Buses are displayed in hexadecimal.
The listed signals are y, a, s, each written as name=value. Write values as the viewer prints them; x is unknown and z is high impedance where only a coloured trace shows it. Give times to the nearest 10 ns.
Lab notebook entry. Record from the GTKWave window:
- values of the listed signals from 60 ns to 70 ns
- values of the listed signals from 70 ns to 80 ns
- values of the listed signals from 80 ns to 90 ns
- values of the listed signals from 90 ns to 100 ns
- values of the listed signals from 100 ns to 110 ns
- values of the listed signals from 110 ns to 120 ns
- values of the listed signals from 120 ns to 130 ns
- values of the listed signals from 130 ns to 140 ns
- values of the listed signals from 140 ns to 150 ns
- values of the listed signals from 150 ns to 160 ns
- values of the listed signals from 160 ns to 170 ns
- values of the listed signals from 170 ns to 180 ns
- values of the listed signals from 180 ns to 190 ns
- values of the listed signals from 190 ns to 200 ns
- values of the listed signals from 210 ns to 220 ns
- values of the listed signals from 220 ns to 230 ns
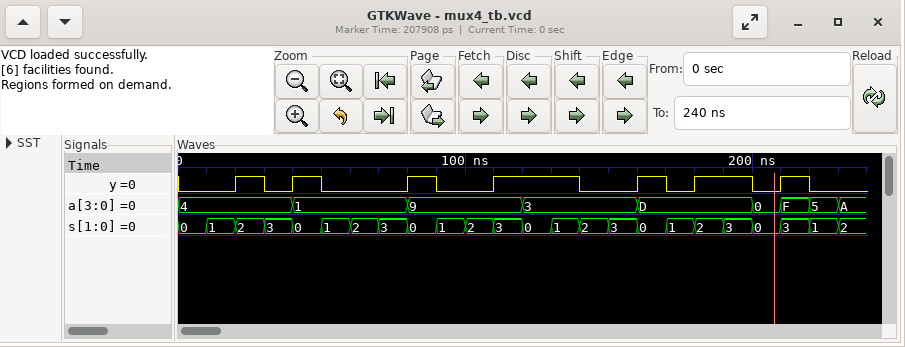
y=0, a=1, s=2
y=0, a=1, s=3
y=1, a=9, s=0
y=0, a=9, s=1
y=0, a=9, s=2
y=1, a=9, s=3
y=1, a=3, s=0
y=1, a=3, s=1
y=0, a=3, s=2
y=0, a=3, s=3
y=1, a=D, s=0
y=0, a=D, s=1
y=1, a=D, s=2
y=1, a=D, s=3
y=1, a=F, s=3
y=0, a=5, s=1
